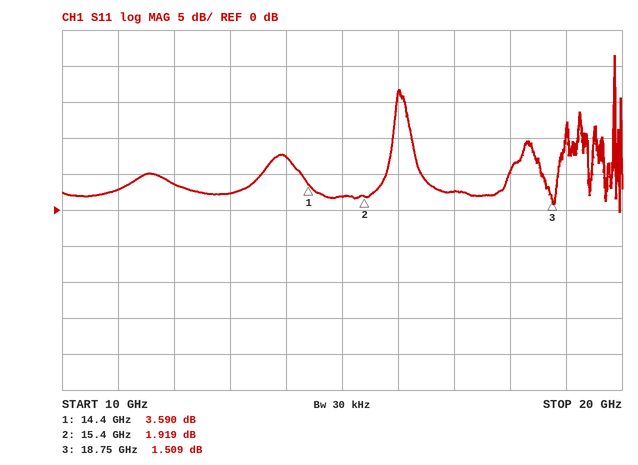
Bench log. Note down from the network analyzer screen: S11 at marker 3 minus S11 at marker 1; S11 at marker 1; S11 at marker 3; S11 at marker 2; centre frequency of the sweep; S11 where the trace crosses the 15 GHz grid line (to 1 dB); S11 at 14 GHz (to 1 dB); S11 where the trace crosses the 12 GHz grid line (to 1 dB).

-2.081 dB
3.590 dB
1.509 dB
1.919 dB
15 GHz
2 dB
7 dB
4 dB
